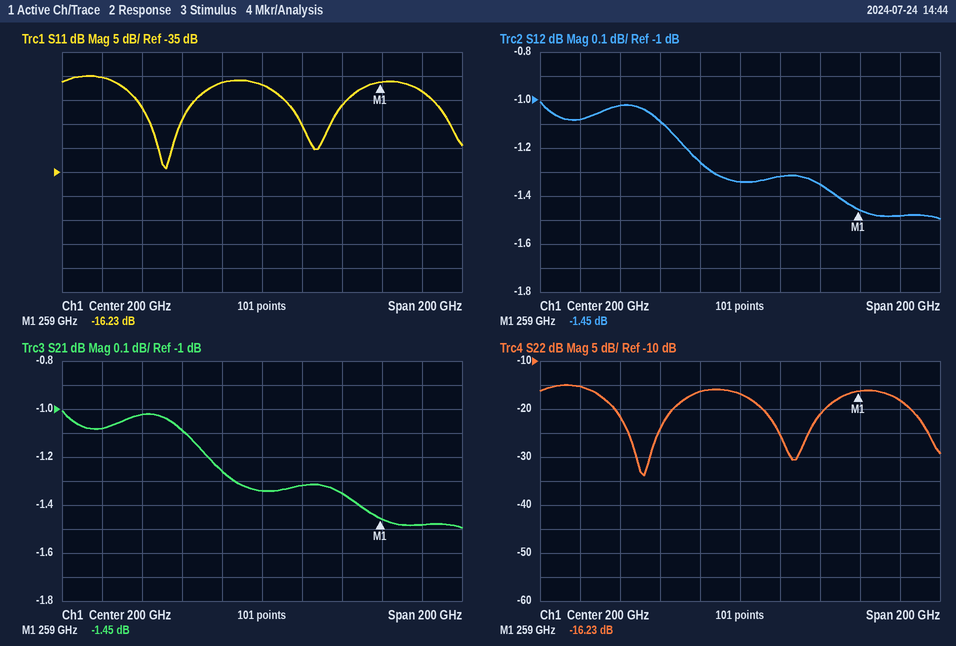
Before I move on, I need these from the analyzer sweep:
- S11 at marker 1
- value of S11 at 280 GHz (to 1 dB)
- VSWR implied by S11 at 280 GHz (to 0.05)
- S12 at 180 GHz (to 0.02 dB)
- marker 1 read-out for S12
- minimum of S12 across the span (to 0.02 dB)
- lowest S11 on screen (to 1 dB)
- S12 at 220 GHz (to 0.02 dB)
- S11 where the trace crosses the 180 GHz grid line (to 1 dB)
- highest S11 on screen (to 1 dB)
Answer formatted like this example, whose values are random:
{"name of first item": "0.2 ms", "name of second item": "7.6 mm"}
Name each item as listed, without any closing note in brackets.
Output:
{"S11 at marker 1": "-16.23 dB", "value of S11 at 280 GHz": "-18 dB", "VSWR implied by S11 at 280 GHz": "1.30", "S12 at 180 GHz": "-1.26 dB", "marker 1 read-out for S12": "-1.45 dB", "minimum of S12 across the span": "-1.50 dB", "lowest S11 on screen": "-34 dB", "S12 at 220 GHz": "-1.32 dB", "S11 where the trace crosses the 180 GHz grid line": "-16 dB", "highest S11 on screen": "-15 dB"}
